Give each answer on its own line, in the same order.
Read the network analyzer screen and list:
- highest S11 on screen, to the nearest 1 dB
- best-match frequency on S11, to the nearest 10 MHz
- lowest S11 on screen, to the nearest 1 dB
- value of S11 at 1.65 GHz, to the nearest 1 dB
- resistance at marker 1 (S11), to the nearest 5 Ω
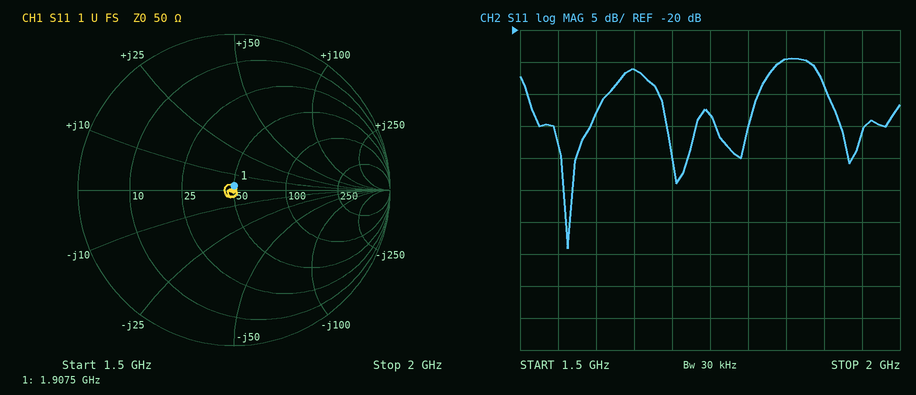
-24 dB
1.56 GHz
-54 dB
-26 dB
50 Ω
